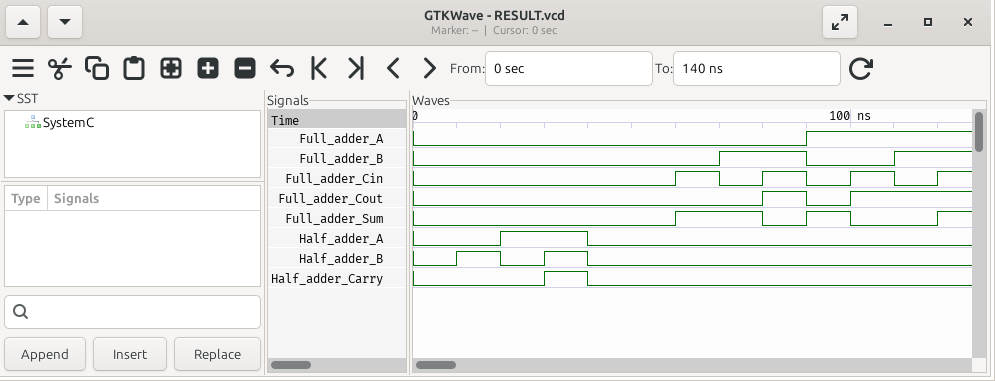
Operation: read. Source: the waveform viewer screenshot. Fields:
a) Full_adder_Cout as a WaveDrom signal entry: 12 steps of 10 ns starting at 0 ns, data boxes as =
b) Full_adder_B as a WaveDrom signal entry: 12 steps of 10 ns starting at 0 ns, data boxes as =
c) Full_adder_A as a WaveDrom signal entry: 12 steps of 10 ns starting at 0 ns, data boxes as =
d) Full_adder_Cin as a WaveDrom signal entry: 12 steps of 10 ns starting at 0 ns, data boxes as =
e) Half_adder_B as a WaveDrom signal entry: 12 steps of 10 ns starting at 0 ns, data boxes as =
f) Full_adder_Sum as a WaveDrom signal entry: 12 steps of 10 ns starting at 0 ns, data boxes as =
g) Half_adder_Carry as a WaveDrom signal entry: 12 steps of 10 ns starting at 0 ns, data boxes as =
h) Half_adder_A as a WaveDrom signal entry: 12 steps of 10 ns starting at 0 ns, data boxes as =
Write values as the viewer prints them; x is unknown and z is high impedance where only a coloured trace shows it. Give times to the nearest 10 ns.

{name: 'Full_adder_Cout', wave: '0.......101.'}
{name: 'Full_adder_B', wave: '0......1.0.1'}
{name: 'Full_adder_A', wave: '0........1..'}
{name: 'Full_adder_Cin', wave: '0.....101010'}
{name: 'Half_adder_B', wave: '01010.......'}
{name: 'Full_adder_Sum', wave: '0.....1.010.'}
{name: 'Half_adder_Carry', wave: '0..10.......'}
{name: 'Half_adder_A', wave: '0.1.0.......'}
